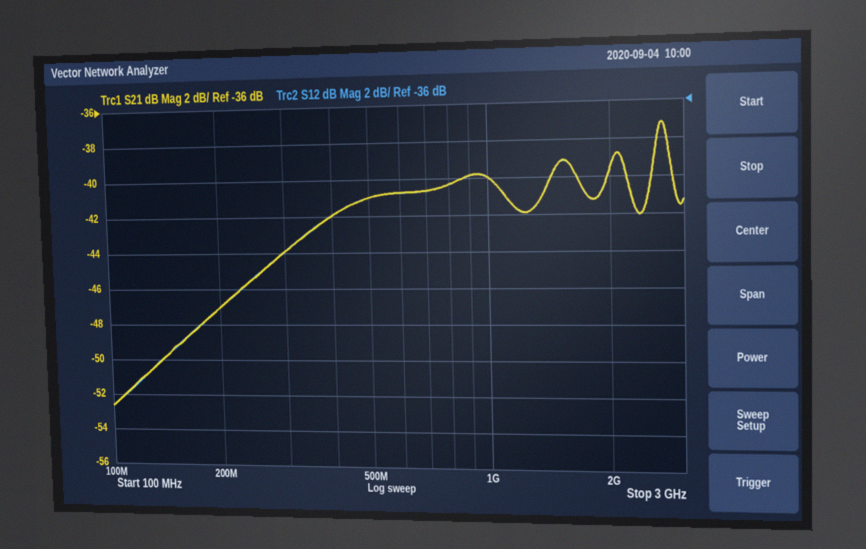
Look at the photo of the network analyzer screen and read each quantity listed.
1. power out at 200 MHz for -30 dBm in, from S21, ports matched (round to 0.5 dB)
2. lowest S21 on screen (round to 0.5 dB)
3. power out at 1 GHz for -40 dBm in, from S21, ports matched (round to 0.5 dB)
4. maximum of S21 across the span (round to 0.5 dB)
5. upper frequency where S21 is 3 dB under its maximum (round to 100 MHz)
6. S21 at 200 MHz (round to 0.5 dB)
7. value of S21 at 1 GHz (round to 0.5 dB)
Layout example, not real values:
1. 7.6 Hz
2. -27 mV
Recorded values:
1. -77.0 dBm
2. -52.5 dB
3. -80.0 dBm
4. -37.0 dB
5. 2.8 GHz
6. -47.0 dB
7. -40.0 dB
